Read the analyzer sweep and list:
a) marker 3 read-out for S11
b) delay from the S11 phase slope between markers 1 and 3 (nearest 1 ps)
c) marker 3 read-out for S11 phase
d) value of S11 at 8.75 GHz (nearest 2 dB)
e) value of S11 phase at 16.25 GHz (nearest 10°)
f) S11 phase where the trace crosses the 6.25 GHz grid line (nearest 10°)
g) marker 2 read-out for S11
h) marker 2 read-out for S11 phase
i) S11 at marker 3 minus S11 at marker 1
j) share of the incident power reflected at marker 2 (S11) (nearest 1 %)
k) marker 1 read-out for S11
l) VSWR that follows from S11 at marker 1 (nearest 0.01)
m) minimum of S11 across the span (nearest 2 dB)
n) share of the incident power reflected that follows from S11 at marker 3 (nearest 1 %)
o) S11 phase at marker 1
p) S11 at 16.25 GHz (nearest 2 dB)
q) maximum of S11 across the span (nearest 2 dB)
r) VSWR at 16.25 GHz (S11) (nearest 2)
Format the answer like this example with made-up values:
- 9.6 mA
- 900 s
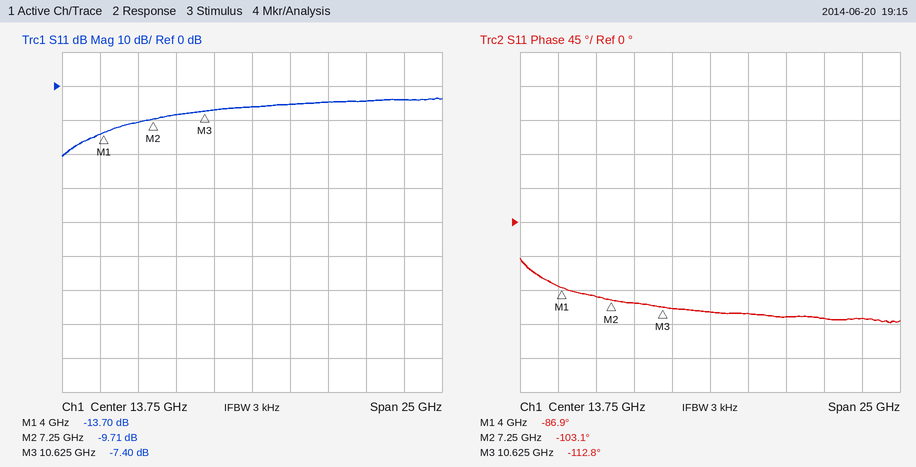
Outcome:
- -7.40 dB
- 11 ps
- -112.8°
- -8 dB
- -120°
- -100°
- -9.71 dB
- -103.1°
- 6.30 dB
- 11 %
- -13.70 dB
- 1.52
- -20 dB
- 18 %
- -86.9°
- -6 dB
- -4 dB
- 4
